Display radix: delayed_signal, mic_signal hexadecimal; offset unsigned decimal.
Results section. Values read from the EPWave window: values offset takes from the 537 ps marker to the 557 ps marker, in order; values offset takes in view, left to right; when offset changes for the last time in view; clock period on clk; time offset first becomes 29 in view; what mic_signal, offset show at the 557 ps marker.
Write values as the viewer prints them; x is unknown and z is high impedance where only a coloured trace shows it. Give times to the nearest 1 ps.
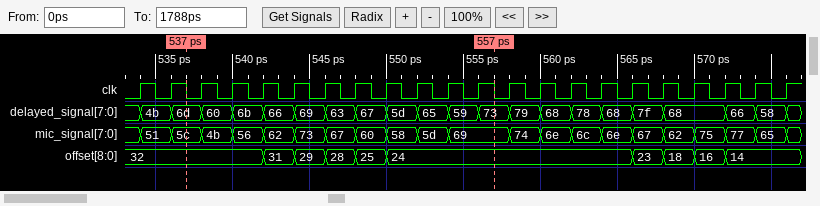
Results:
32, 31, 29, 28, 25, 24
32, 31, 29, 28, 25, 24, 23, 18, 16, 14
572 ps
2 ps
544 ps
mic_signal=69, offset=24
